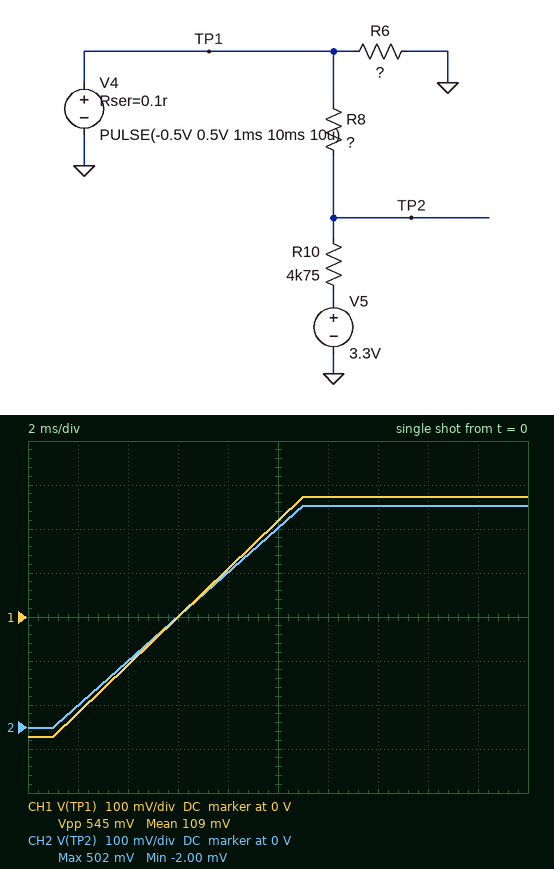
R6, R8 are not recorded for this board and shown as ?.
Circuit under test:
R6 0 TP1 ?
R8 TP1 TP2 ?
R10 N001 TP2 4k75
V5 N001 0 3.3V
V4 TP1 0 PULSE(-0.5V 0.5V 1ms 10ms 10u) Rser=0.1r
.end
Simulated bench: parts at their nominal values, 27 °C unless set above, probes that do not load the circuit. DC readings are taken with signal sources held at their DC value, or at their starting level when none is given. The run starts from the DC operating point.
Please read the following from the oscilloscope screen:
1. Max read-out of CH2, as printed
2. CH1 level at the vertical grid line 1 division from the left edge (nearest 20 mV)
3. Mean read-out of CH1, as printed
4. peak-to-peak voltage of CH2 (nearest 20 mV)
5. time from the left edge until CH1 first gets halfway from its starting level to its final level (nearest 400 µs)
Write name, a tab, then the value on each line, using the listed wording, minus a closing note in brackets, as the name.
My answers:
Max read-out of CH2, as printed	502 mV
CH1 level at the vertical grid line 1 division from the left edge	-220 mV
Mean read-out of CH1, as printed	109 mV
peak-to-peak voltage of CH2	500 mV
time from the left edge until CH1 first gets halfway from its starting level to its final level	6.0 ms
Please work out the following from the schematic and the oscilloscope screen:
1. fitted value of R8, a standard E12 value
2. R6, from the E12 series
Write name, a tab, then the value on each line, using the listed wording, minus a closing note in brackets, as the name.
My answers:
fitted value of R8, a standard E12 value	390 Ω
R6, from the E12 series	0.12 Ω
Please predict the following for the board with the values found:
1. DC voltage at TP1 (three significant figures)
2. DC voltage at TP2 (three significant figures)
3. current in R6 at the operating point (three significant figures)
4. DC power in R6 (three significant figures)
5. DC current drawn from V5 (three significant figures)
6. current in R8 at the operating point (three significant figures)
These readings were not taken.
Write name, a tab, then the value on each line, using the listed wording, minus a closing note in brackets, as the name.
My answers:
DC voltage at TP1	-273 mV
DC voltage at TP2	-1.61 mV
current in R6 at the operating point	2.27 A
DC power in R6	620 mW
DC current drawn from V5	695 µA
current in R8 at the operating point	695 µA
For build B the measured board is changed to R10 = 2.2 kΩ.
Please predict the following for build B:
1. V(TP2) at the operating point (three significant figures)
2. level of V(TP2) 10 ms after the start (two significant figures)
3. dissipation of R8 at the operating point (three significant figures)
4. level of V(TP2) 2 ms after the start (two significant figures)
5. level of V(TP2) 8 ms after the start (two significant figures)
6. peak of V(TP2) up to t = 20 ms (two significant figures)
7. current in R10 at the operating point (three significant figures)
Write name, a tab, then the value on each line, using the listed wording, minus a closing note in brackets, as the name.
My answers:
V(TP2) at the operating point	265 mV
level of V(TP2) 10 ms after the start	680 mV
dissipation of R8 at the operating point	742 µW
level of V(TP2) 2 ms after the start	310 mV
level of V(TP2) 8 ms after the start	590 mV
peak of V(TP2) up to t = 20 ms	730 mV
current in R10 at the operating point	1.38 mA
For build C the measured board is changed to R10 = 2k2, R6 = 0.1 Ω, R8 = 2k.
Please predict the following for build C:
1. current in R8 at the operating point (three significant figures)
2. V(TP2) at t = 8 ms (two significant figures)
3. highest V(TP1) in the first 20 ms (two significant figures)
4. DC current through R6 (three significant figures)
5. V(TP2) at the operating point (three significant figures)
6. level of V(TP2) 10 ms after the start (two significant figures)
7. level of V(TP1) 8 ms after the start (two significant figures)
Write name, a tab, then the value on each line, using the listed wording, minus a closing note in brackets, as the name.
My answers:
current in R8 at the operating point	845 µA
V(TP2) at t = 8 ms	1.6 V
highest V(TP1) in the first 20 ms	250 mV
DC current through R6	2.50 A
V(TP2) at the operating point	1.44 V
level of V(TP2) 10 ms after the start	1.7 V
level of V(TP1) 8 ms after the start	100 mV
